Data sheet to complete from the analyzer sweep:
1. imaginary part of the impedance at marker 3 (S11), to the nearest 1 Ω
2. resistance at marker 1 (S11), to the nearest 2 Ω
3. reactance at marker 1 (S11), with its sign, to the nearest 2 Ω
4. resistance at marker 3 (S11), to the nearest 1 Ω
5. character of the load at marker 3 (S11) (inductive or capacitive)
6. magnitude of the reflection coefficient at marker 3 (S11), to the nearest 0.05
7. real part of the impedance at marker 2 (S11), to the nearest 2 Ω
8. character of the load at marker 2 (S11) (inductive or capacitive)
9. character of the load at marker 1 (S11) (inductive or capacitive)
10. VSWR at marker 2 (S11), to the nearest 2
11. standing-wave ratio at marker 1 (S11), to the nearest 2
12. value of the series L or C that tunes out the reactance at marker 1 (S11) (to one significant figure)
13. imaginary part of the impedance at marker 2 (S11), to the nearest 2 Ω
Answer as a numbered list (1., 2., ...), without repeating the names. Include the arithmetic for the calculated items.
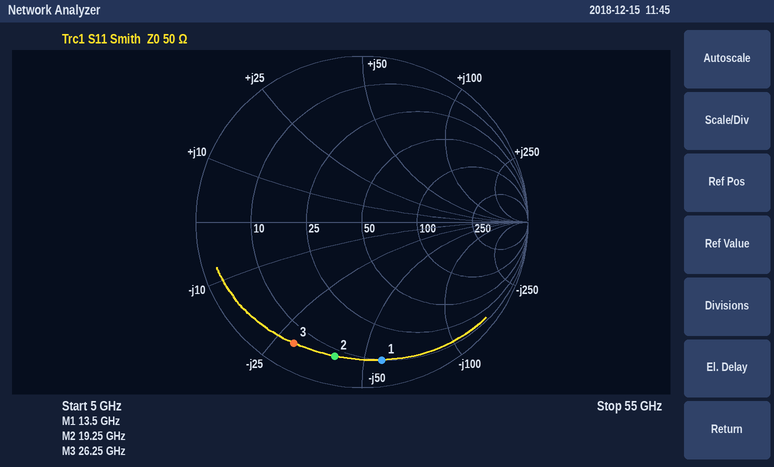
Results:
1. -29 Ω
2. 10 Ω
3. -56 Ω
4. 6 Ω
5. capacitive
6. 0.85
7. 8 Ω
8. capacitive
9. capacitive
10. 10
11. 12
12. L = 56 Ω/(2π × 13.5 GHz) ≈ 660 pH, so 700 pH to one significant figure
13. -40 Ω
